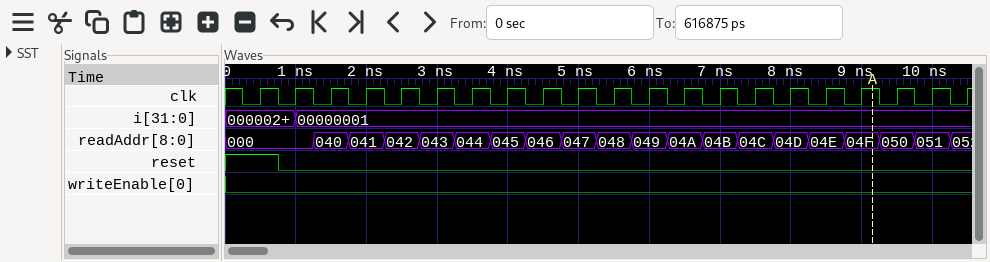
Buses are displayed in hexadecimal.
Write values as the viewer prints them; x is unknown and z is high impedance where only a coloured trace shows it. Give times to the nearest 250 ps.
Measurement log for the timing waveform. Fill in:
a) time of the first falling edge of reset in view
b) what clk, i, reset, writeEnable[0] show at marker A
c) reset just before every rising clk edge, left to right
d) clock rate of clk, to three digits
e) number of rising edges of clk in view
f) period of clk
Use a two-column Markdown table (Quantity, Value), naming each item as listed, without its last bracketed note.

| Quantity | Value |
|---|---|
| time of the first falling edge of reset in view | 750 ps |
| what clk, i, reset, writeEnable[0] show at marker A | clk=1, i=00000001, reset=0, writeEnable[0]=0 |
| reset just before every rising clk edge, left to right | 1 0 0 0 0 0 0 0 0 0 0 0 0 0 0 0 0 0 0 0 0 |
| clock rate of clk, to three digits | 2.00 GHz |
| number of rising edges of clk in view | 21 |
| period of clk | 500 ps |
